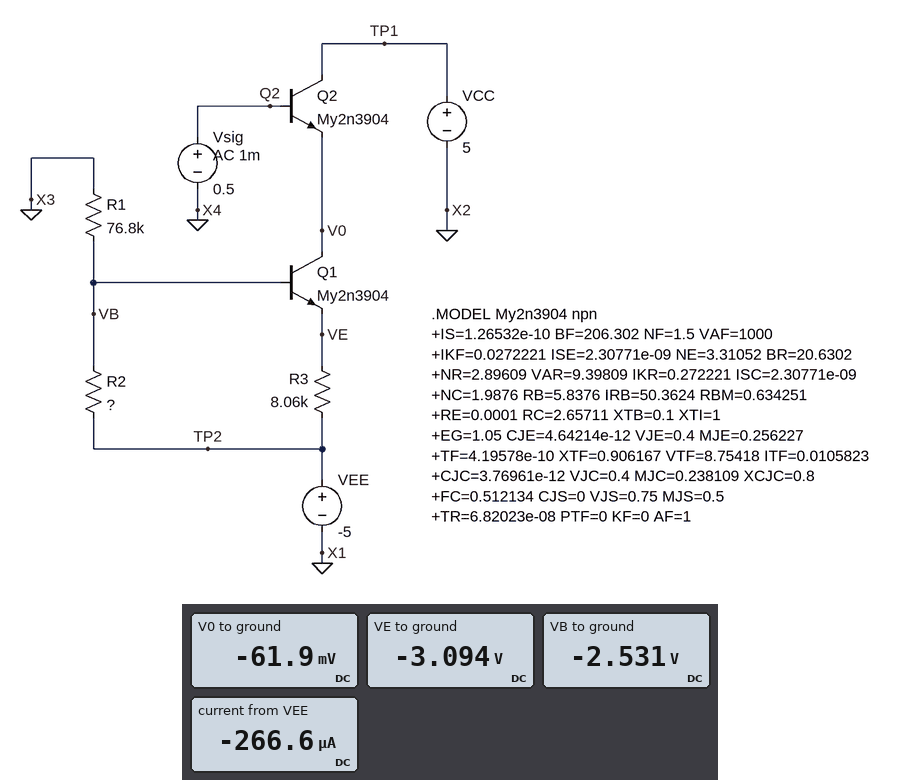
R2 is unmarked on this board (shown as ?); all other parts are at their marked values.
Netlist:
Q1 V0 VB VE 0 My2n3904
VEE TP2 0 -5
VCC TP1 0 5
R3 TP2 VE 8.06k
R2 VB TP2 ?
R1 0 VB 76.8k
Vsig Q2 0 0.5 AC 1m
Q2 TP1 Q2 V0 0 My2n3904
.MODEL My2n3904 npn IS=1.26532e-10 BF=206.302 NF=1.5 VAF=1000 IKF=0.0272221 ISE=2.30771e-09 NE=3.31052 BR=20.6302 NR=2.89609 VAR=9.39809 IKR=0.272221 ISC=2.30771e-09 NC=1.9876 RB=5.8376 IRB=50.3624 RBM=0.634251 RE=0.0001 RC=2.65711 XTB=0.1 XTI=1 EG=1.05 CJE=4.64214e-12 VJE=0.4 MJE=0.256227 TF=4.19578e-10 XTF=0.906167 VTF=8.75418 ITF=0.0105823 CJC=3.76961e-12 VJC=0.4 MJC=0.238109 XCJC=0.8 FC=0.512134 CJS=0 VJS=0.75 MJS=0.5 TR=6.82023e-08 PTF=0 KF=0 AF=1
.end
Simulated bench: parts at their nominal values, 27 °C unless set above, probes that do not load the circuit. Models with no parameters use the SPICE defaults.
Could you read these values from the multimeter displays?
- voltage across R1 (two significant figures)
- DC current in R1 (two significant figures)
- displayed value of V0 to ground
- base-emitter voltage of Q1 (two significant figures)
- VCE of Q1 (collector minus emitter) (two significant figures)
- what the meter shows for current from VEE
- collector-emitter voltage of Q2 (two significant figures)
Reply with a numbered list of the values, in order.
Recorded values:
1. 2.5 V
2. 33 µA
3. -61.9 mV
4. 560 mV
5. 3.0 V
6. -266.6 µA
7. 5.1 V
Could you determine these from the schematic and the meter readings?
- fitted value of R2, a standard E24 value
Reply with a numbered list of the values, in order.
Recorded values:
1. 82 kΩ
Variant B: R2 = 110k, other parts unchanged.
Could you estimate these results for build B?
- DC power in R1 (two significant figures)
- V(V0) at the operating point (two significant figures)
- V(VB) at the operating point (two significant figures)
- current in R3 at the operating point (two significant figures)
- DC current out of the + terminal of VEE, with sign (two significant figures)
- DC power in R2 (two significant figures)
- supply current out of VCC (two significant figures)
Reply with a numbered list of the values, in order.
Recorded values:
1. 63 µW
2. -68 mV
3. -2.2 V
4. 280 µA
5. -300 µA
6. 71 µW
7. 270 µA
